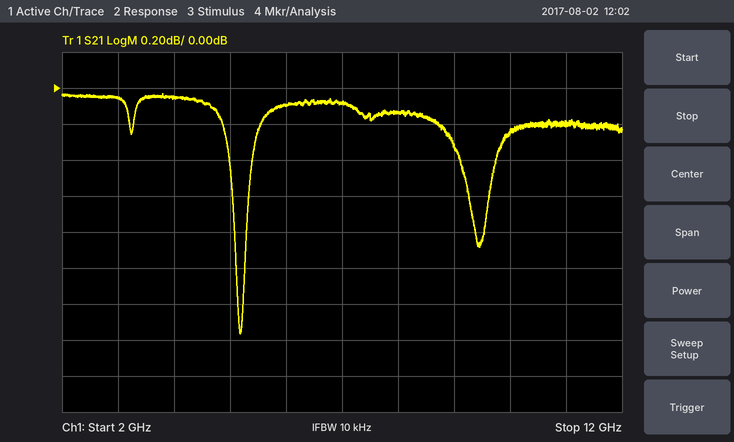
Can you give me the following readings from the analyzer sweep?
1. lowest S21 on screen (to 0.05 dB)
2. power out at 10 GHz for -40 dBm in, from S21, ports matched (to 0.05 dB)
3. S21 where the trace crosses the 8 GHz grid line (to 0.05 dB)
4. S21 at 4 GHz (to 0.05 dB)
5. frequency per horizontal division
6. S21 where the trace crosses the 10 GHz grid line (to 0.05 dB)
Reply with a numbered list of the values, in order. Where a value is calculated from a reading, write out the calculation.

1. -1.35 dB
2. -40 dBm + (-0.25 dB) = -40.25 dBm
3. -0.15 dB
4. -0.05 dB
5. 1 GHz
6. -0.25 dB
